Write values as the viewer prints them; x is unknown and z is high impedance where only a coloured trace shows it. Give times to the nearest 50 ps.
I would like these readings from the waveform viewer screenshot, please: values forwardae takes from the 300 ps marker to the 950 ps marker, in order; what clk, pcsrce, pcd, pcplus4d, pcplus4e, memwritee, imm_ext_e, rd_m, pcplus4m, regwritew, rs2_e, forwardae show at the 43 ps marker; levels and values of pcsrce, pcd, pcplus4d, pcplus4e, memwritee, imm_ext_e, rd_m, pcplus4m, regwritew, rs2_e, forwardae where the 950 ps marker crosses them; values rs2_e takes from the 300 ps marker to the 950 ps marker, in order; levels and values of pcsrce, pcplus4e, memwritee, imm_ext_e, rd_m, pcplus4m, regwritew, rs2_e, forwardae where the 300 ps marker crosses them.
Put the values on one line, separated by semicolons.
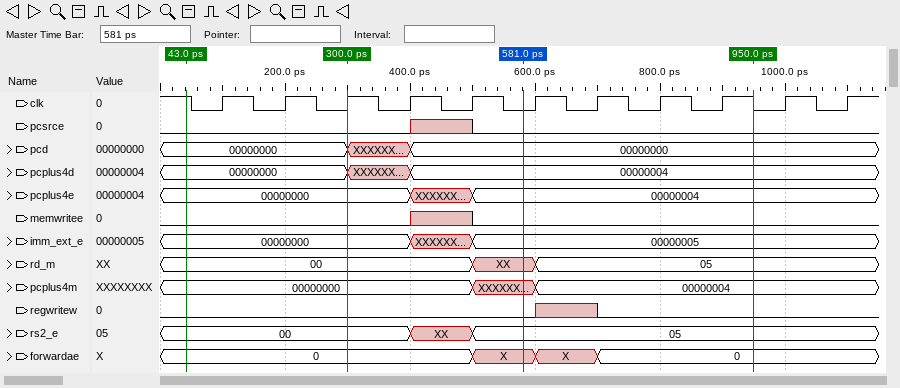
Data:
0, X, X, 0; clk=1, pcsrce=0, pcd=00000000, pcplus4d=00000000, pcplus4e=00000000, memwritee=0, imm_ext_e=00000000, rd_m=00, pcplus4m=00000000, regwritew=0, rs2_e=00, forwardae=0; pcsrce=0, pcd=00000000, pcplus4d=00000004, pcplus4e=00000004, memwritee=0, imm_ext_e=00000005, rd_m=05, pcplus4m=00000004, regwritew=0, rs2_e=05, forwardae=0; 00, XX, 05; pcsrce=0, pcplus4e=00000000, memwritee=0, imm_ext_e=00000000, rd_m=00, pcplus4m=00000000, regwritew=0, rs2_e=00, forwardae=0
